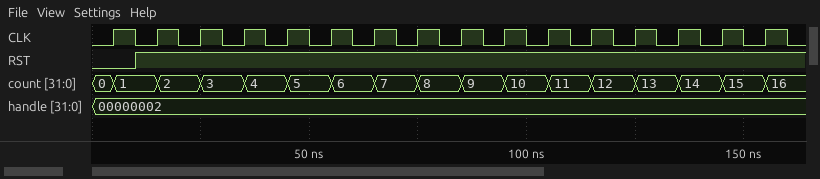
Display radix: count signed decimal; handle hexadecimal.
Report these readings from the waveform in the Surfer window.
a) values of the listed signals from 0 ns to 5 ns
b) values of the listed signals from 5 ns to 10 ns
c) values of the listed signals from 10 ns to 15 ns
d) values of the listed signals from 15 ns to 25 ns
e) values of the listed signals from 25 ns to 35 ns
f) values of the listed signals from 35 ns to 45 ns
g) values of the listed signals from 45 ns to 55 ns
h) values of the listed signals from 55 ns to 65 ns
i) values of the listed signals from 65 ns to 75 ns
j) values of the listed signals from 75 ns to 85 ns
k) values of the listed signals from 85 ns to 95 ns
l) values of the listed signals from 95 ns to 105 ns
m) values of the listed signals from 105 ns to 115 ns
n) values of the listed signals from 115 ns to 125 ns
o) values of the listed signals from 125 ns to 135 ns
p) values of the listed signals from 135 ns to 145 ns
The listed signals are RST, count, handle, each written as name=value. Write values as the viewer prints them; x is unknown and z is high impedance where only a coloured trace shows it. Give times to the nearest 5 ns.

RST=0, count=0, handle=00000002
RST=0, count=1, handle=00000002
RST=1, count=1, handle=00000002
RST=1, count=2, handle=00000002
RST=1, count=3, handle=00000002
RST=1, count=4, handle=00000002
RST=1, count=5, handle=00000002
RST=1, count=6, handle=00000002
RST=1, count=7, handle=00000002
RST=1, count=8, handle=00000002
RST=1, count=9, handle=00000002
RST=1, count=10, handle=00000002
RST=1, count=11, handle=00000002
RST=1, count=12, handle=00000002
RST=1, count=13, handle=00000002
RST=1, count=14, handle=00000002
